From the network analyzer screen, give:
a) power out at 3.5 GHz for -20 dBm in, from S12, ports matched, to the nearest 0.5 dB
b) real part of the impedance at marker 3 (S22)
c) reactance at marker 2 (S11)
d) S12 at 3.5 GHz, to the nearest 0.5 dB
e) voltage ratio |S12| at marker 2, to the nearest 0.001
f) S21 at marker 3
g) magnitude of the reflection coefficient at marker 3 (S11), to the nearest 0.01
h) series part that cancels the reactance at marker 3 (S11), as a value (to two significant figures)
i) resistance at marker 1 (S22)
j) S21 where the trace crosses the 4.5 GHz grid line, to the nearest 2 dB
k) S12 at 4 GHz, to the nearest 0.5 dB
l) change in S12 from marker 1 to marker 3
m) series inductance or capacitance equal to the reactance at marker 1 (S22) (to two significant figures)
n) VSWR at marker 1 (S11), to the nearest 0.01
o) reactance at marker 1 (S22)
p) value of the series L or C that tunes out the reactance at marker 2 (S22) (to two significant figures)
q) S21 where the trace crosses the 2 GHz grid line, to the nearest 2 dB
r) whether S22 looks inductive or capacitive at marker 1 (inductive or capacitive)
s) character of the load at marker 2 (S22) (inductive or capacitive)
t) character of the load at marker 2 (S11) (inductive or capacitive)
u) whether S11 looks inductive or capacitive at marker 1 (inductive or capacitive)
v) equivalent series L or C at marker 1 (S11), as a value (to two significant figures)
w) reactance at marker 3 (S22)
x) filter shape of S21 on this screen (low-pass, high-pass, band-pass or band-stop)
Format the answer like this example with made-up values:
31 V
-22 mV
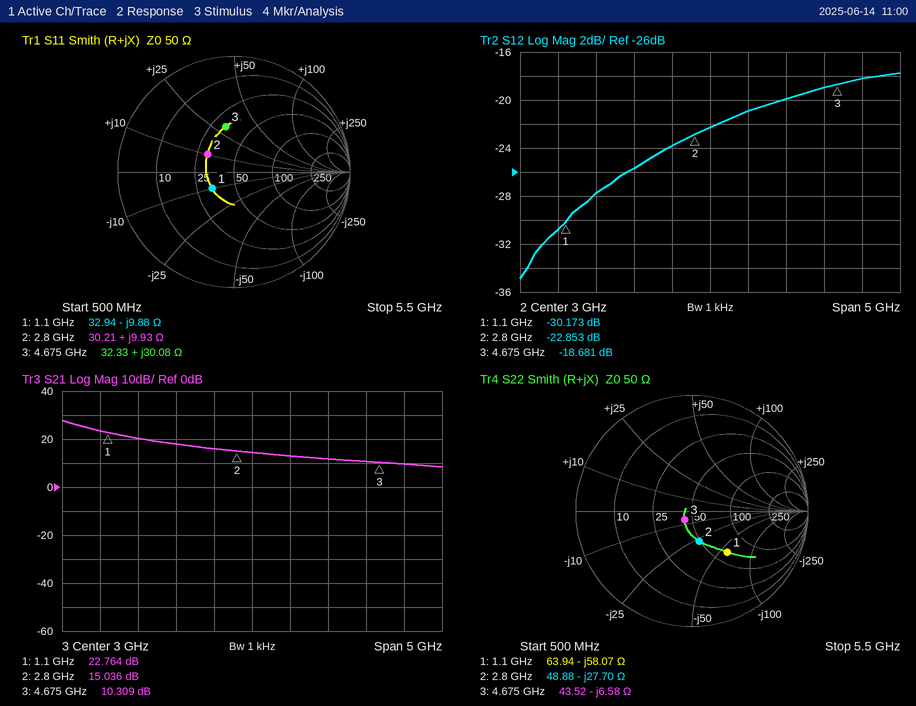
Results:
-41.0 dBm
43.52 Ω
+9.93 Ω
-21.0 dB
0.072
10.309 dB
0.40
1.1 pF
63.94 Ω
10 dB
-20.0 dB
11.492 dB
2.5 pF
1.62
-58.07 Ω
1.6 nH
18 dB
capacitive
capacitive
inductive
capacitive
15 pF
-6.58 Ω
low-pass
